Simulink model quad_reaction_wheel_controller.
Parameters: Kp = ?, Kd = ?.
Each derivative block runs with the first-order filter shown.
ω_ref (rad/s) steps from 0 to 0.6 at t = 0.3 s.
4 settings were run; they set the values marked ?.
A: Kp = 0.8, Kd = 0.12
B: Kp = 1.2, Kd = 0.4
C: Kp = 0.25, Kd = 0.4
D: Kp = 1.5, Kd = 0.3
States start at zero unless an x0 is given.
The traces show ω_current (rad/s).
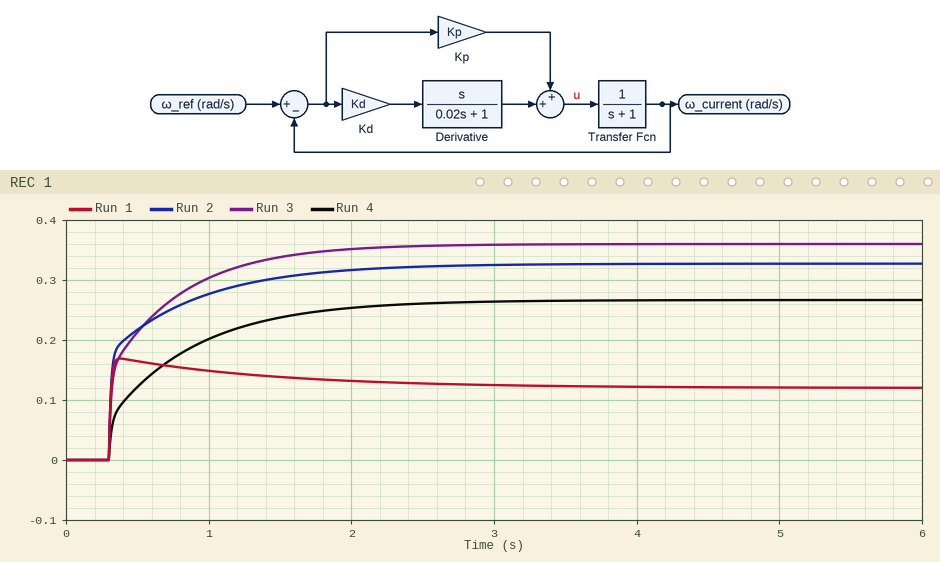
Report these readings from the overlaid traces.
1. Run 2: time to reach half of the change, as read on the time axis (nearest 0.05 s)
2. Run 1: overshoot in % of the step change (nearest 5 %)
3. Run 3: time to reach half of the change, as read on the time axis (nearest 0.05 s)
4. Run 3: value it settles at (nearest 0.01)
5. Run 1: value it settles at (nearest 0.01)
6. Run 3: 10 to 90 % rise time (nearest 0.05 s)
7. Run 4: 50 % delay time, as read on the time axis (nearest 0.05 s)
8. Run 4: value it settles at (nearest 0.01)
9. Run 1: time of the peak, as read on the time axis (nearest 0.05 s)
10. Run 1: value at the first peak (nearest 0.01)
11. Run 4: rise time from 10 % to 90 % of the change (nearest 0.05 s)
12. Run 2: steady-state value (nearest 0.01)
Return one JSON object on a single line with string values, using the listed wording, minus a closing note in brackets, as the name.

{"Run 2: time to reach half of the change, as read on the time axis": "0.35 s", "Run 1: overshoot in % of the step change": "40 %", "Run 3: time to reach half of the change, as read on the time axis": "0.40 s", "Run 3: value it settles at": "0.36", "Run 1: value it settles at": "0.12", "Run 3: 10 to 90 % rise time": "0.95 s", "Run 4: 50 % delay time, as read on the time axis": "0.55 s", "Run 4: value it settles at": "0.27", "Run 1: time of the peak, as read on the time axis": "0.40 s", "Run 1: value at the first peak": "0.17", "Run 4: rise time from 10 % to 90 % of the change": "1.25 s", "Run 2: steady-state value": "0.33"}
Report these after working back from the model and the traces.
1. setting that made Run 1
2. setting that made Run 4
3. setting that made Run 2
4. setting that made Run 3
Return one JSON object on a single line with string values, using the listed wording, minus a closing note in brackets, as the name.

{"setting that made Run 1": "C", "setting that made Run 4": "A", "setting that made Run 2": "B", "setting that made Run 3": "D"}
